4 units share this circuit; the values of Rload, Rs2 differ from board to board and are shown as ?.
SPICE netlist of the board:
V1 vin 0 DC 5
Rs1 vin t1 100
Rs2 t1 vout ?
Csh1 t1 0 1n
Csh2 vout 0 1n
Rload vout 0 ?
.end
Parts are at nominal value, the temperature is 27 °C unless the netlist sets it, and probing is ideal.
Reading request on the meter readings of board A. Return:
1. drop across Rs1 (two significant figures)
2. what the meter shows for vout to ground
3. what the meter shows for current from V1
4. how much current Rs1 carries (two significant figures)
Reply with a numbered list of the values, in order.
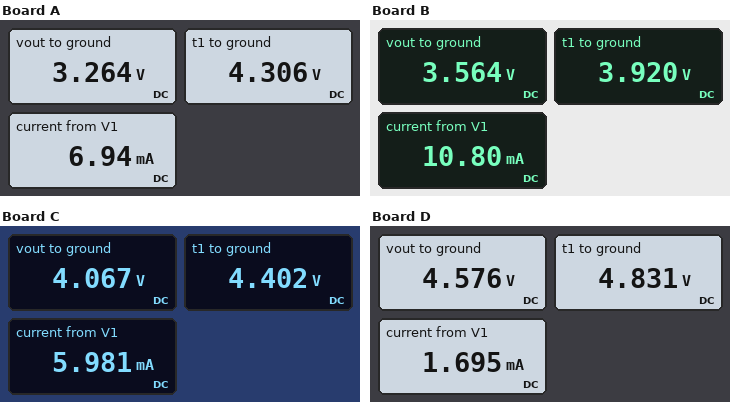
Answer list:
1. 690 mV
2. 3.264 V
3. 6.94 mA
4. 6.9 mA
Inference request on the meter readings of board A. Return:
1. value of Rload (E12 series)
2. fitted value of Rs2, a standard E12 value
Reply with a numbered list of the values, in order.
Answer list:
1. 470 Ω
2. 150 Ω
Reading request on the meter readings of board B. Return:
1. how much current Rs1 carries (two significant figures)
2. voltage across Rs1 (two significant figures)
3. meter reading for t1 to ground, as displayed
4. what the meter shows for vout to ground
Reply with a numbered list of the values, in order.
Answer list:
1. 11 mA
2. 1.1 V
3. 3.920 V
4. 3.564 V
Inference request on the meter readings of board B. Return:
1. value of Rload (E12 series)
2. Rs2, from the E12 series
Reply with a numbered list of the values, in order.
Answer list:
1. 330 Ω
2. 33 Ω
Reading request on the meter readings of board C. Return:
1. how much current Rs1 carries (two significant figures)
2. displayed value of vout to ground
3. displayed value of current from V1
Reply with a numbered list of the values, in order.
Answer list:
1. 6.0 mA
2. 4.067 V
3. 5.981 mA
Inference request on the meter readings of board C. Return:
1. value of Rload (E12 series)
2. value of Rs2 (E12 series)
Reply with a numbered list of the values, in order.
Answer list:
1. 680 Ω
2. 56 Ω
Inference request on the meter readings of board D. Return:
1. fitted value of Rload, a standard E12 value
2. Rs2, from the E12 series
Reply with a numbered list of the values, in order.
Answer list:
1. 2.7 kΩ
2. 150 Ω
